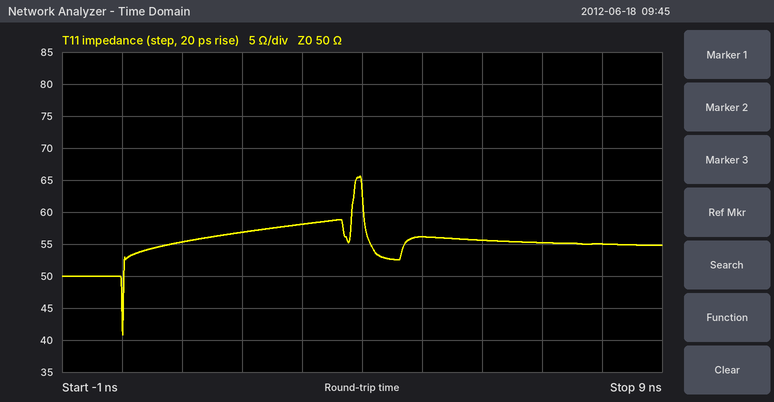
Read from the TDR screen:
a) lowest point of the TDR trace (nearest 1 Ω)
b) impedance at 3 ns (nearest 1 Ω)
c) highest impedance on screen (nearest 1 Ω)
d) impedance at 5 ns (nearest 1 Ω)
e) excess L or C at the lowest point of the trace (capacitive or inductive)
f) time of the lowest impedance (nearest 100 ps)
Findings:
41 Ω
58 Ω
66 Ω
56 Ω
capacitive
0.0 ns
